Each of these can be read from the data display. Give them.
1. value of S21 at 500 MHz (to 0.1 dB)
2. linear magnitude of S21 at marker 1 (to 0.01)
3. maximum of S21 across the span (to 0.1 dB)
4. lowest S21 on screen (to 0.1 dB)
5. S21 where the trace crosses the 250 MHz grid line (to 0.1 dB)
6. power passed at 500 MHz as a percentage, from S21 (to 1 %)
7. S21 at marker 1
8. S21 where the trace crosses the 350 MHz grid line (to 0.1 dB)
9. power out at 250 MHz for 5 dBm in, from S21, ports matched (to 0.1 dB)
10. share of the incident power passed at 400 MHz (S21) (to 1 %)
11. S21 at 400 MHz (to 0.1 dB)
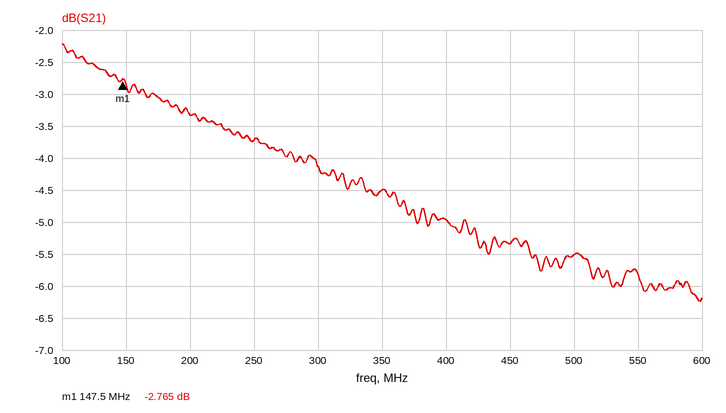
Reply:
-5.5 dB
0.73
-2.2 dB
-6.2 dB
-3.7 dB
28 %
-2.765 dB
-4.5 dB
1.3 dBm
32 %
-5.0 dB
